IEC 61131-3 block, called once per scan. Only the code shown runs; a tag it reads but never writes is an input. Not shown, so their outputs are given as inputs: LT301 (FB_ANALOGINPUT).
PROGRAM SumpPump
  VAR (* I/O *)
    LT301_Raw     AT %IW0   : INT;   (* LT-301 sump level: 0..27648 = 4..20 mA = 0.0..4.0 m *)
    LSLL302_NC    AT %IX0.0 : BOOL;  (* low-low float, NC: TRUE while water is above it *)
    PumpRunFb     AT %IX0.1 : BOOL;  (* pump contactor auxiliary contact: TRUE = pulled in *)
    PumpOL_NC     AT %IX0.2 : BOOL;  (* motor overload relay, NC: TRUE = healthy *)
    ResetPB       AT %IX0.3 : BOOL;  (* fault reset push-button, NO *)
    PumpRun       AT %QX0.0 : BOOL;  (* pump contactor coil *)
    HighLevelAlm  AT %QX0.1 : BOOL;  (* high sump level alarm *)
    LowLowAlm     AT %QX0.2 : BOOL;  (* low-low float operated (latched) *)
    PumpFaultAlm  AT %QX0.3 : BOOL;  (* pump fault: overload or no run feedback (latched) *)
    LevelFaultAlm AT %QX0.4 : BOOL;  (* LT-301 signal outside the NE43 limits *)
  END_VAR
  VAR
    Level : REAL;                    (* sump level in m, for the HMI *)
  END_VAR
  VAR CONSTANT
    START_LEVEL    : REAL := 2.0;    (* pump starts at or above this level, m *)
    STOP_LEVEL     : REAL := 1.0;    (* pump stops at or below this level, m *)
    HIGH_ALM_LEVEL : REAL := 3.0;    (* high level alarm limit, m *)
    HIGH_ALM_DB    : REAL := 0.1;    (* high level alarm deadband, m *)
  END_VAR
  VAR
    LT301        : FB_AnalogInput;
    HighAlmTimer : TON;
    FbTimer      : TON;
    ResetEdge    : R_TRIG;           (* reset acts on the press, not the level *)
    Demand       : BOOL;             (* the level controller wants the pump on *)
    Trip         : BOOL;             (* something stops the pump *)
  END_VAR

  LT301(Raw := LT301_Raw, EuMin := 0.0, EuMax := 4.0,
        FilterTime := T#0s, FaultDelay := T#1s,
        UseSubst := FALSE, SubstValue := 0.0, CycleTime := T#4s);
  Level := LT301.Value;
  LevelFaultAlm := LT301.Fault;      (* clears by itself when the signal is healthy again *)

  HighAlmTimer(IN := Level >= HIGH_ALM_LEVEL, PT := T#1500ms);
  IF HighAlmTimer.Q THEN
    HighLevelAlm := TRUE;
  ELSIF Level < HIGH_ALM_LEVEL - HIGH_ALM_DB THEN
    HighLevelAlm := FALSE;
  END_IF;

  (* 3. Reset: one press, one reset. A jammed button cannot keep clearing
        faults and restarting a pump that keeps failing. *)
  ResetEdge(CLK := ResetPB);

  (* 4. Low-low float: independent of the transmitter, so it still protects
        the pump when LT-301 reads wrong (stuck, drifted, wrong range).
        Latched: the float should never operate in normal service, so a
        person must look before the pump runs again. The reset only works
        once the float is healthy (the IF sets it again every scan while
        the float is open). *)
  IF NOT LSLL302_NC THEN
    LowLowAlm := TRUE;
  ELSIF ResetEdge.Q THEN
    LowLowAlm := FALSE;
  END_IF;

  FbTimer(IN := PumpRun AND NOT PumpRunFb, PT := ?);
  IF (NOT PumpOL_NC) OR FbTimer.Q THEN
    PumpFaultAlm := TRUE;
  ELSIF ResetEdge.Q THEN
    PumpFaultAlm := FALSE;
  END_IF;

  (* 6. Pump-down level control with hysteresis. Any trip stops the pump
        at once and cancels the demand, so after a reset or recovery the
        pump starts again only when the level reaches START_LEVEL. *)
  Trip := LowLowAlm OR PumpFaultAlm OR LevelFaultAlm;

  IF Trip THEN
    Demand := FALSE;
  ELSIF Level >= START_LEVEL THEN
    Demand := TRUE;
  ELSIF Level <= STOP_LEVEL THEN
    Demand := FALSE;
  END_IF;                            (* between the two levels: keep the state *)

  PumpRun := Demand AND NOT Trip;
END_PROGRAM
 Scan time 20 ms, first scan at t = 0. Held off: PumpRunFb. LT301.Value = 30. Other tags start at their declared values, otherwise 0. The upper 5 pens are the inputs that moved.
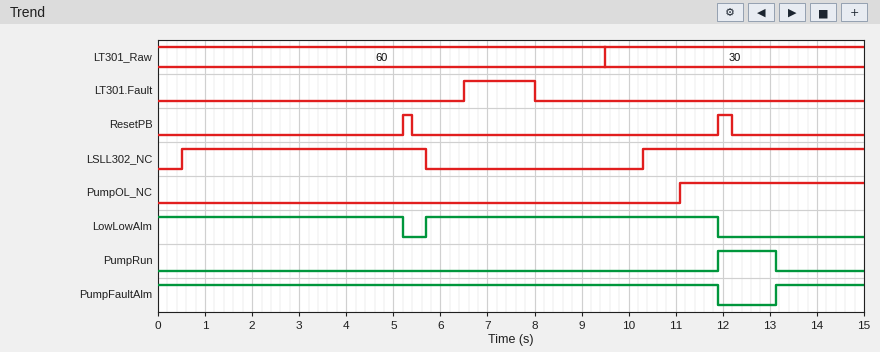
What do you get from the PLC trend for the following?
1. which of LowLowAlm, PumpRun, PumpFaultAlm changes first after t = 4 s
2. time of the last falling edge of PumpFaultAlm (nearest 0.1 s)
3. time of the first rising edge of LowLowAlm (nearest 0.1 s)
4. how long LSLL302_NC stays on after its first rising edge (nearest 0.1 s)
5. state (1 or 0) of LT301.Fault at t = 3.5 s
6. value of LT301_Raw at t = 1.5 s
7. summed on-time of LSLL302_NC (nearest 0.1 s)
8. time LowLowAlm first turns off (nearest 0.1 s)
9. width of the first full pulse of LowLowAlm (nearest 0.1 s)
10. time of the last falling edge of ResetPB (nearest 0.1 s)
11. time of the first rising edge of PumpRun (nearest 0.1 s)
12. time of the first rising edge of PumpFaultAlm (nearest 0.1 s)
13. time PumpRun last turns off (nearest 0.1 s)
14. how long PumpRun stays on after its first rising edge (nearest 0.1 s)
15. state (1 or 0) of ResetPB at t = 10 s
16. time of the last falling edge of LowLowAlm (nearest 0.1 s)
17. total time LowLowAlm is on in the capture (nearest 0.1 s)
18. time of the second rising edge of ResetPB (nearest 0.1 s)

LowLowAlm
11.9 s
5.7 s
5.2 s
0
60
9.9 s
5.2 s
6.2 s
12.2 s
11.9 s
13.1 s
13.1 s
1.2 s
0
11.9 s
11.4 s
11.9 s
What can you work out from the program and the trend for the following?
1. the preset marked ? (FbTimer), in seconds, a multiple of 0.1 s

1.2 s
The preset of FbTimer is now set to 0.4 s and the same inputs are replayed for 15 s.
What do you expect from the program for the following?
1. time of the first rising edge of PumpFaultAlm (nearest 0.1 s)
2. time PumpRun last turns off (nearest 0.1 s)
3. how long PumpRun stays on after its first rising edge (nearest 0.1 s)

12.3 s
12.3 s
0.4 s
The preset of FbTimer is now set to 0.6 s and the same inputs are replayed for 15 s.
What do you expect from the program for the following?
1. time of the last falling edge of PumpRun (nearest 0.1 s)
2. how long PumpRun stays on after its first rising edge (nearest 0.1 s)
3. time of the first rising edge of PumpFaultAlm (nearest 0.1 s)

12.5 s
0.6 s
12.5 s
